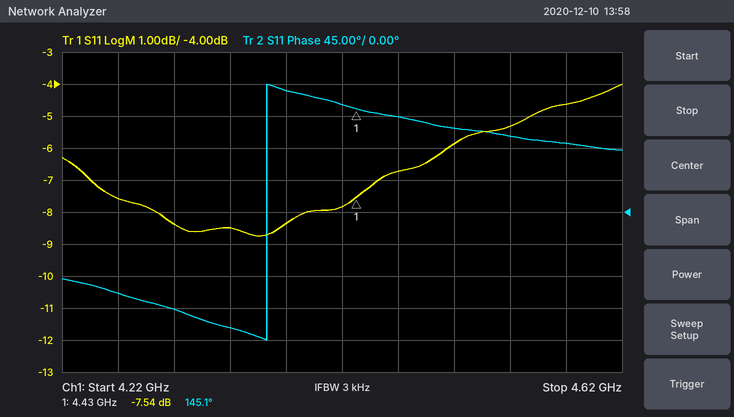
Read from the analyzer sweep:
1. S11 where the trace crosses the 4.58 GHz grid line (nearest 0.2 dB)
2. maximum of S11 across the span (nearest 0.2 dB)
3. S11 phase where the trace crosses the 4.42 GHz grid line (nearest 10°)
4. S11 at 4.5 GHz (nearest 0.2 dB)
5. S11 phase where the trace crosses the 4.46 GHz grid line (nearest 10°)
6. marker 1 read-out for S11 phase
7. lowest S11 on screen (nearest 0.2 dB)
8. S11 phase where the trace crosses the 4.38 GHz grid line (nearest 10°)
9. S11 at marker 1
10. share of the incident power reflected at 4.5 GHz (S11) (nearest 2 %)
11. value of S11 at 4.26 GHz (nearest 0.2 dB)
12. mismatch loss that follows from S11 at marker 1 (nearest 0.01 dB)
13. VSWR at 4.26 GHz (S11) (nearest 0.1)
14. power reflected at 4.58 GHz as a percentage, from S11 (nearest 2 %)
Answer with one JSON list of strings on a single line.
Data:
["-4.6 dB", "-4.0 dB", "150°", "-5.8 dB", "130°", "145.1°", "-8.8 dB", "170°", "-7.54 dB", "26 %", "-7.6 dB", "0.84 dB", "2.4", "34 %"]
